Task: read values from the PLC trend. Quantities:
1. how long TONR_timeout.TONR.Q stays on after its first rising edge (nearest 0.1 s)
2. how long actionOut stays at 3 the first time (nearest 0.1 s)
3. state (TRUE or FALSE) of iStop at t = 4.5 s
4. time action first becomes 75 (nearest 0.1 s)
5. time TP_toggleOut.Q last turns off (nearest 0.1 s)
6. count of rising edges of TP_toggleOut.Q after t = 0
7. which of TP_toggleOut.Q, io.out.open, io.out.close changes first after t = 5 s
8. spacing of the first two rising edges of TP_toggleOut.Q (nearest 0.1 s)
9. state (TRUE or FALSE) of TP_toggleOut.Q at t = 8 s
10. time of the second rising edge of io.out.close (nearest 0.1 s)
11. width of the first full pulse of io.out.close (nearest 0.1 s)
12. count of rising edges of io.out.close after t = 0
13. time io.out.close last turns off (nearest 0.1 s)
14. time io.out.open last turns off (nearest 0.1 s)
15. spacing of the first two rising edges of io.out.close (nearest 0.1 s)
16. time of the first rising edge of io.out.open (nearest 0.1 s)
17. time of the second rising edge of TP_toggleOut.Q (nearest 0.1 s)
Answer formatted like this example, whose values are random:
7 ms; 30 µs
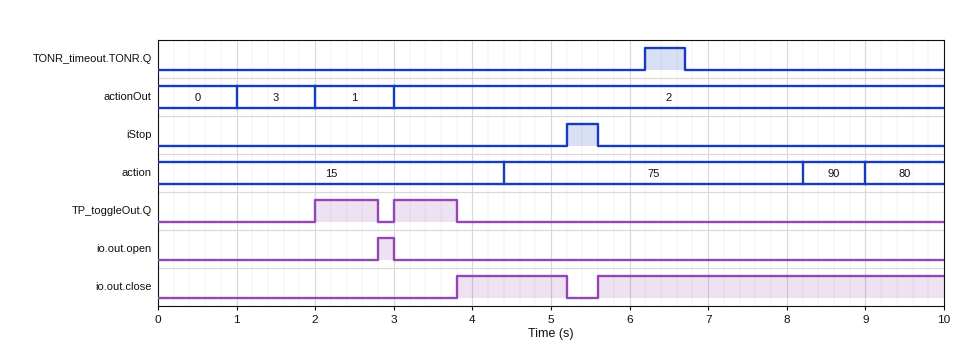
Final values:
0.5 s; 1.0 s; FALSE; 4.4 s; 3.8 s; 2; io.out.close; 1.0 s; FALSE; 5.6 s; 1.4 s; 2; 5.2 s; 3.0 s; 1.8 s; 2.8 s; 3.0 s
